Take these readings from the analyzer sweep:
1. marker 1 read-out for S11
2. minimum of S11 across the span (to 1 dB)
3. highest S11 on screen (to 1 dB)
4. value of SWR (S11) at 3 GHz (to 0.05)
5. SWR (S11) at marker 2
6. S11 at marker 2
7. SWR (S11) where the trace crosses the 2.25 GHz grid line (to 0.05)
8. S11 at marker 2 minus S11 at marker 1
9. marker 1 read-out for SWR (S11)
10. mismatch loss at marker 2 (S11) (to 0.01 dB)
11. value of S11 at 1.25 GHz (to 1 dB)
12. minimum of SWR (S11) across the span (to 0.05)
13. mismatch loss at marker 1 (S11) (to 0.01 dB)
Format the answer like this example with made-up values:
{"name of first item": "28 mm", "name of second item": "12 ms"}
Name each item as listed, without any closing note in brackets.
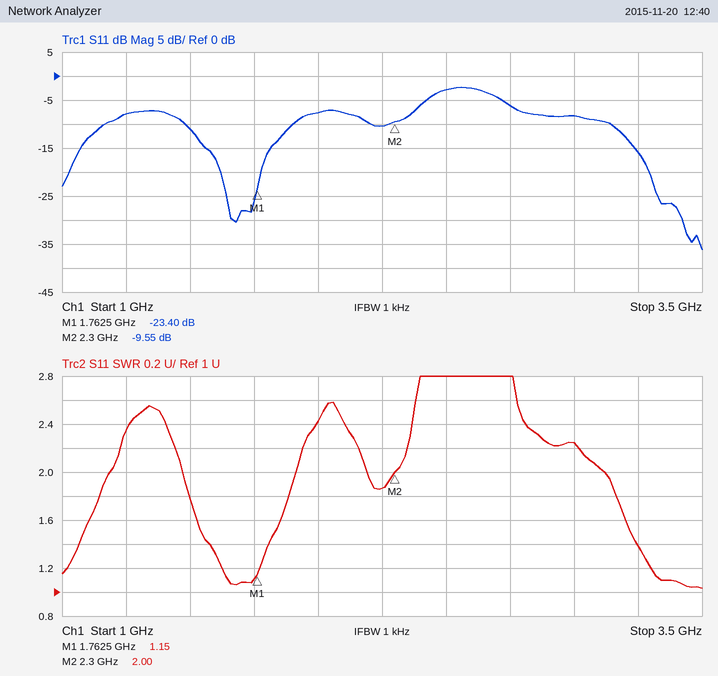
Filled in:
{"marker 1 read-out for S11": "-23.40 dB", "minimum of S11 across the span": "-36 dB", "highest S11 on screen": "-2 dB", "value of SWR (S11) at 3 GHz": "2.25", "SWR (S11) at marker 2": "2.00", "S11 at marker 2": "-9.55 dB", "SWR (S11) where the trace crosses the 2.25 GHz grid line": "1.85", "S11 at marker 2 minus S11 at marker 1": "13.85 dB", "marker 1 read-out for SWR": "1.15", "mismatch loss at marker 2 (S11)": "0.51 dB", "value of S11 at 1.25 GHz": "-8 dB", "minimum of SWR (S11) across the span": "1.05", "mismatch loss at marker 1 (S11)": "0.02 dB"}
